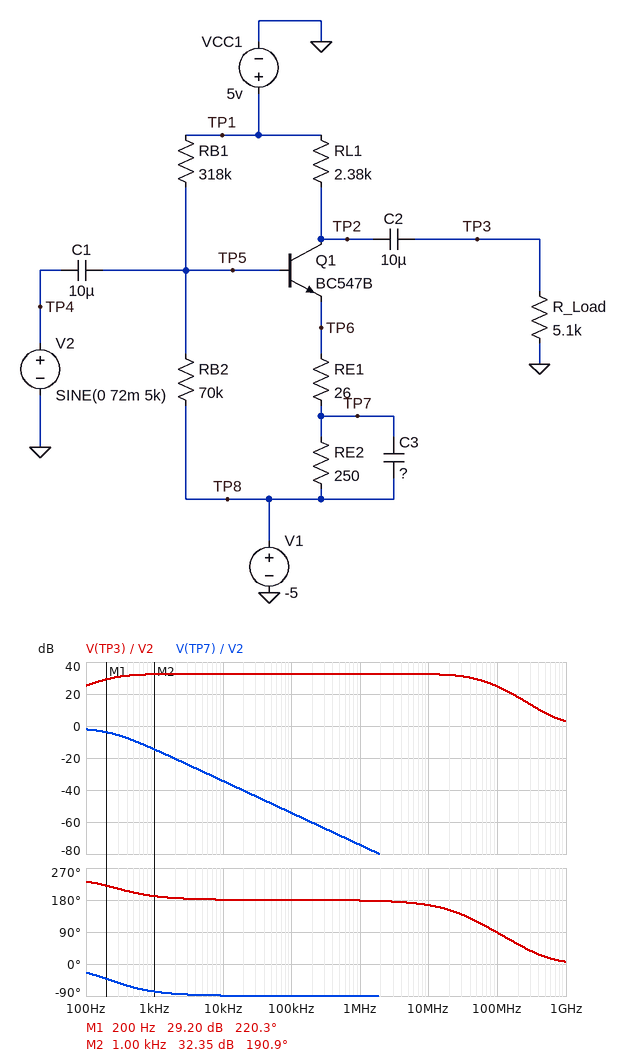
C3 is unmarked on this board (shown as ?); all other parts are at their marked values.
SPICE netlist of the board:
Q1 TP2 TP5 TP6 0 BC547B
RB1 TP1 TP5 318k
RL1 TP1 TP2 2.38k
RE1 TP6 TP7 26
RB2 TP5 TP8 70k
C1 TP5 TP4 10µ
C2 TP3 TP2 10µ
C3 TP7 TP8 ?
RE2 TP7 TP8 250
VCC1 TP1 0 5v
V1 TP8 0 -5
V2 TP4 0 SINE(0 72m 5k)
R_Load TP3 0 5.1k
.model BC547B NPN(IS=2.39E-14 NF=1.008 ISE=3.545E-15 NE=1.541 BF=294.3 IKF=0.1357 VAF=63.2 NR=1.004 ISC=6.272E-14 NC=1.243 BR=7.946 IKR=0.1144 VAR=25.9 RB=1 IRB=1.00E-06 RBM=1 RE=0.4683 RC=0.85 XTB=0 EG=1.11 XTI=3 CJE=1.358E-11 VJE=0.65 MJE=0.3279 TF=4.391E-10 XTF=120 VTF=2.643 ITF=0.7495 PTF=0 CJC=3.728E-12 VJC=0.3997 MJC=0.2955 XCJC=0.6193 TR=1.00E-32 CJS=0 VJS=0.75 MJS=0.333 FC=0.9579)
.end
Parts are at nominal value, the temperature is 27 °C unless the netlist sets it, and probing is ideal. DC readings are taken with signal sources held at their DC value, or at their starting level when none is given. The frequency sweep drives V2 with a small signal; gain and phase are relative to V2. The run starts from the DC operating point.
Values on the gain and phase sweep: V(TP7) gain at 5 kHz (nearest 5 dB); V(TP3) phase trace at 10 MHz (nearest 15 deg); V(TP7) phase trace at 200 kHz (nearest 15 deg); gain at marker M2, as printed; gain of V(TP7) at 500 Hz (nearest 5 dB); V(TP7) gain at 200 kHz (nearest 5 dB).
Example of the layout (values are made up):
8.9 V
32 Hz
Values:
-30 dB
165 deg
-90 deg
32.35 dB
-10 dB
-60 dB
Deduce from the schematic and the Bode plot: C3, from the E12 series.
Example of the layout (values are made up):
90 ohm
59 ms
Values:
22 µF
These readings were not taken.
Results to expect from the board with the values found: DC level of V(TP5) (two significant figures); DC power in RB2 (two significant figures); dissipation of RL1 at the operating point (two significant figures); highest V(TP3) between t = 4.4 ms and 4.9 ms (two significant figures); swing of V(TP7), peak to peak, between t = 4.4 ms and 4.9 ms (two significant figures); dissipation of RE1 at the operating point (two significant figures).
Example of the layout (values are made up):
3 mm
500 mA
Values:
-3.7 V
25 µW
14 mW
2.7 V
5.3 mV
150 µW
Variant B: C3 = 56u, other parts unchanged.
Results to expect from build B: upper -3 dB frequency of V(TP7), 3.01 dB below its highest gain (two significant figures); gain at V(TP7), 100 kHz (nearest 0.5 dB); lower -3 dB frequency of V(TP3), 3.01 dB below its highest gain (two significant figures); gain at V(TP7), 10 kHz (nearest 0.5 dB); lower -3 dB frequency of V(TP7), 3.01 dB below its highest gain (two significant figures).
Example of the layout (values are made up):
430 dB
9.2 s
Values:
88 Hz
-62.5 dB
86 Hz
-42.5 dB
470 mHz
